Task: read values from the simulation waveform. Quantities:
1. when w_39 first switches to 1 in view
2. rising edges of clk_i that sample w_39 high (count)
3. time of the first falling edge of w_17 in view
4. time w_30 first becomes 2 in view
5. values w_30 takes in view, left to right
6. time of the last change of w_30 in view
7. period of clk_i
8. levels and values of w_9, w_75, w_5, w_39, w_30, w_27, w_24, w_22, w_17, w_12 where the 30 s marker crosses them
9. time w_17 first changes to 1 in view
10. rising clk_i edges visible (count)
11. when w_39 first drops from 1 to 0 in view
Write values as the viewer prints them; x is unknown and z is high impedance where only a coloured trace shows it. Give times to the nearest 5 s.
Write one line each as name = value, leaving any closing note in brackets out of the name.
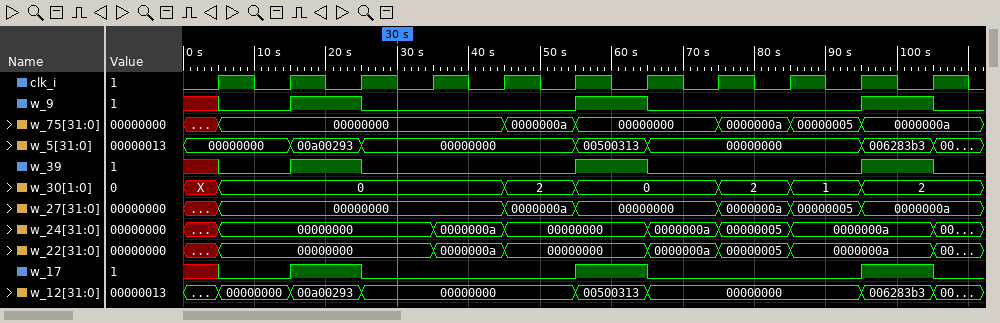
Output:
when w_39 first switches to 1 in view = 15 s
rising edges of clk_i that sample w_39 high = 3
time of the first falling edge of w_17 in view = 25 s
time w_30 first becomes 2 in view = 45 s
values w_30 takes in view, left to right = X, 0, 2, 0, 2, 1, 2
time of the last change of w_30 in view = 95 s
period of clk_i = 10 s
levels and values of w_9, w_75, w_5, w_39, w_30, w_27, w_24, w_22, w_17, w_12 where the 30 s marker crosses them = w_9=0, w_75=00000000, w_5=00000000, w_39=0, w_30=0, w_27=00000000, w_24=00000000, w_22=00000000, w_17=0, w_12=00000000
time w_17 first changes to 1 in view = 15 s
rising clk_i edges visible = 11
when w_39 first drops from 1 to 0 in view = 25 s
